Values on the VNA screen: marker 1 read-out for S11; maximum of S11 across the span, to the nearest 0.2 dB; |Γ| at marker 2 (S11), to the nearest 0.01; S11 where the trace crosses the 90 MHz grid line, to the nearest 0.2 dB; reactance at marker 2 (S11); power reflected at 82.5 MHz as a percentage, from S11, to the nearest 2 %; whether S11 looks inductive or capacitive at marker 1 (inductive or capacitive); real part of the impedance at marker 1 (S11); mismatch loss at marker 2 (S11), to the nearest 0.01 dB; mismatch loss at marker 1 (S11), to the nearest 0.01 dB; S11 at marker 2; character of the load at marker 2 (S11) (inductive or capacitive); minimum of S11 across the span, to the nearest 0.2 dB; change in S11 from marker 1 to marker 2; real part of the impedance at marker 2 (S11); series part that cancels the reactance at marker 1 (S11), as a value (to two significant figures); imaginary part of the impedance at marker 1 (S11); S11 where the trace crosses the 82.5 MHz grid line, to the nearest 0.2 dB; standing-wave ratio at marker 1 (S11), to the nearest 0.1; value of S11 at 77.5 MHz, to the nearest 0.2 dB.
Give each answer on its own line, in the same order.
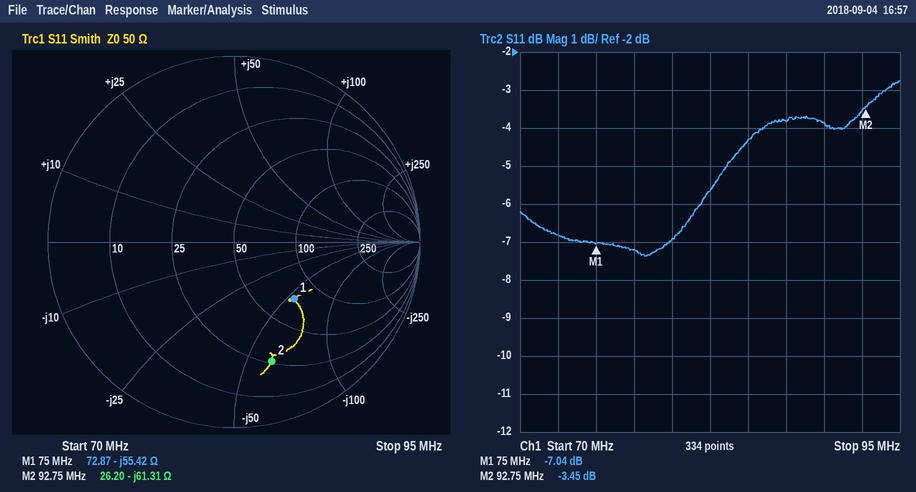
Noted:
-7.04 dB
-2.8 dB
0.67
-3.8 dB
-61.31 Ω
28 %
capacitive
72.87 Ω
2.61 dB
0.96 dB
-3.45 dB
capacitive
-7.4 dB
3.59 dB
26.20 Ω
120 nH
-55.42 Ω
-5.6 dB
2.6
-7.2 dB
